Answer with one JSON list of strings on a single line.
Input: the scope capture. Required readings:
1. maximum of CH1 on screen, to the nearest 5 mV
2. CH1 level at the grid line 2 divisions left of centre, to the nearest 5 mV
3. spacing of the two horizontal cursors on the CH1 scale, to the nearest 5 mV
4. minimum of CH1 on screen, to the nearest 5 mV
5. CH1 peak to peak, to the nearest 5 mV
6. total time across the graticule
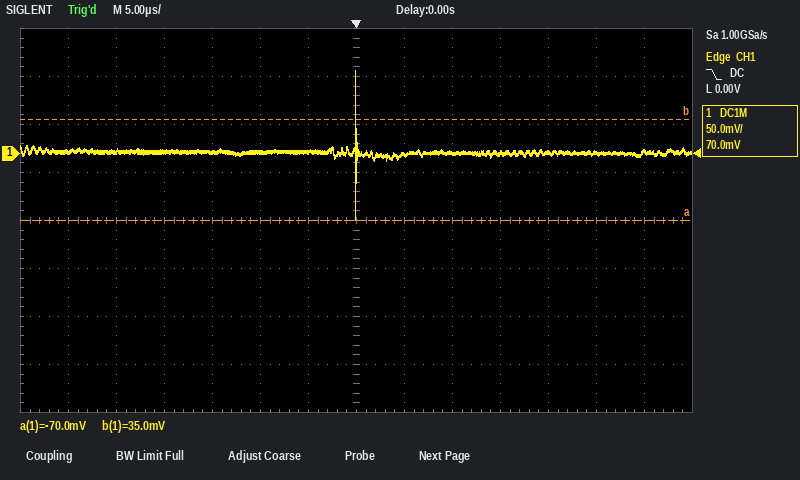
["85 mV", "0 mV", "105 mV", "-70 mV", "155 mV", "70 µs"]
